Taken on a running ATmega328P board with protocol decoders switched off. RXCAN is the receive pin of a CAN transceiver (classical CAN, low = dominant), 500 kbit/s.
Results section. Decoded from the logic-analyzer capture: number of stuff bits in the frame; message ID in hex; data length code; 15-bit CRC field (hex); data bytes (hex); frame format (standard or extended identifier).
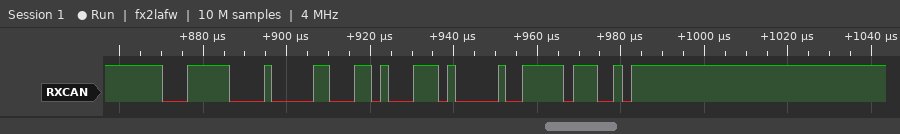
4
0x1F1
2
0x03FC
34 74
standard
